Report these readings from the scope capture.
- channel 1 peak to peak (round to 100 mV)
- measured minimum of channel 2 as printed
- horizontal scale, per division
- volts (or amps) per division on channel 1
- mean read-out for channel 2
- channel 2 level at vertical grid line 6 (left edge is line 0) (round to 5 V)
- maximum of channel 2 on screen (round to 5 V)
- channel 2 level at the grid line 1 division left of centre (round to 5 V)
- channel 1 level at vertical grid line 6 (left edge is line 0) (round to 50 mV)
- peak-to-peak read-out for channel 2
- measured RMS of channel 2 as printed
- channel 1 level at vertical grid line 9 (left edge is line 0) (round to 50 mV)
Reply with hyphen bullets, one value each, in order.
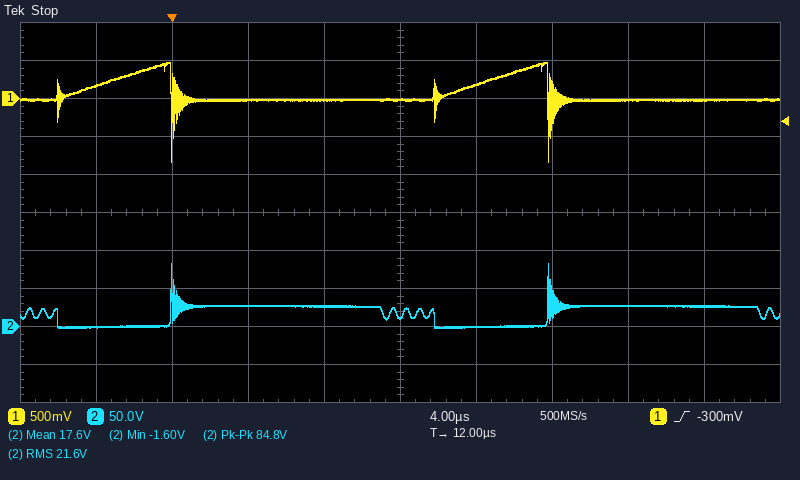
- 1.30 V
- -1.60 V
- 4 µs
- 500 mV
- 17.6 V
- 0 V
- 85 V
- 25 V
- 200 mV
- 84.8 V
- 21.6 V
- 0 mV
